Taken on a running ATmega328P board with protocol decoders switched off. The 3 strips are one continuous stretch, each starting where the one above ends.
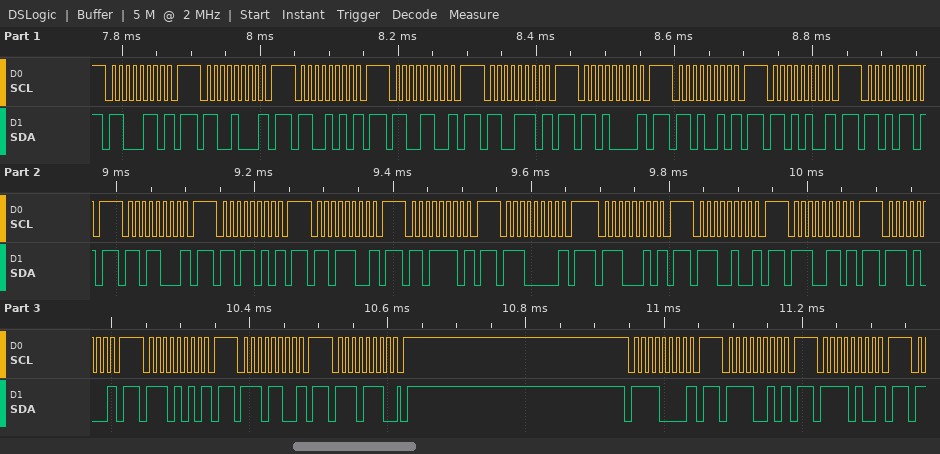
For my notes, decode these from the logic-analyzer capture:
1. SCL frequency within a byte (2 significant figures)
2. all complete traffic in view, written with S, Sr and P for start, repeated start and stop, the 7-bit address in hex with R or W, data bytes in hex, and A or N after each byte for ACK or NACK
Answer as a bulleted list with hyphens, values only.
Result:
- 100 kHz
- S 63W N P S 64W N P S 65W N P S 66W N P S 67W N P S 68W N P S 69W N P S 6AW N P S 6BW N P S 6CW N P S 6DW N P S 6EW N P S 6FW N P S 70W N P S 71W N P S 72W N P S 73W N P S 74W N P S 75W N P S 76W N P S 77W A P S 78W N P S 79W N P S 7AW N P
